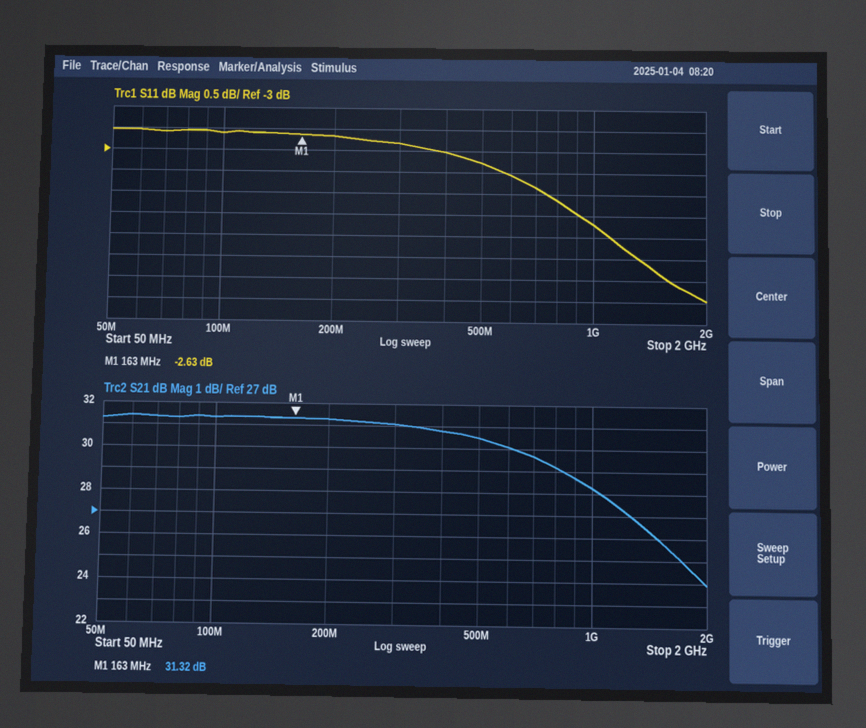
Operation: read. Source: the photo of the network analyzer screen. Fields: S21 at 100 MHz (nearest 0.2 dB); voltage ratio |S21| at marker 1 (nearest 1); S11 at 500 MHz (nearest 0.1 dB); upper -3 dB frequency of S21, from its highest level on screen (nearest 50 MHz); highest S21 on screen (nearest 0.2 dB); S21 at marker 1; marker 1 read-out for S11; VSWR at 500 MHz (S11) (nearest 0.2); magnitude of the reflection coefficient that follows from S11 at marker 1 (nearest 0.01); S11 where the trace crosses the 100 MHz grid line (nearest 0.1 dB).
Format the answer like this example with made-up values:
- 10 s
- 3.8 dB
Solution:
- 31.4 dB
- 37
- -3.3 dB
- 950 MHz
- 31.4 dB
- 31.32 dB
- -2.63 dB
- 5.4
- 0.74
- -2.6 dB
